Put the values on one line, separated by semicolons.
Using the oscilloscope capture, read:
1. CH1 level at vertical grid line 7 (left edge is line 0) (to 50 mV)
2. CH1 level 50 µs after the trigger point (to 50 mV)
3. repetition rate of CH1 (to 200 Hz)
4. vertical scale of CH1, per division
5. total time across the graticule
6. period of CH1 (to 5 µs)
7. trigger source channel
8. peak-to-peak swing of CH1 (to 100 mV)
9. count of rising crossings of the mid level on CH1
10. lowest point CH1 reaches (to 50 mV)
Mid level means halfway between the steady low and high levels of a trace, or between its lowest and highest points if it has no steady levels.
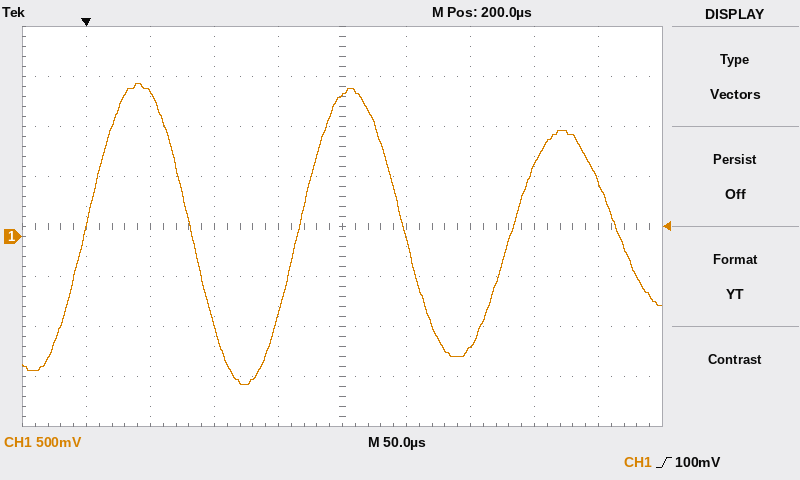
-1.10 V; 1.45 V; 6.0 kHz; 500 mV; 500 µs; 165 µs; CH1; 3.00 V; 3; -1.50 V
